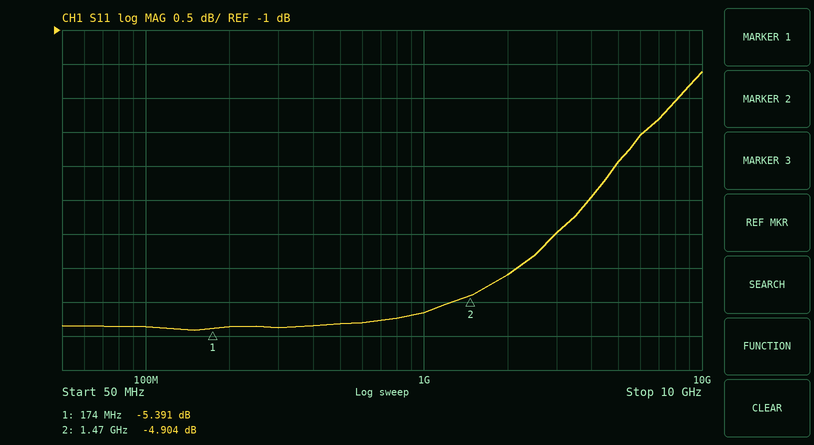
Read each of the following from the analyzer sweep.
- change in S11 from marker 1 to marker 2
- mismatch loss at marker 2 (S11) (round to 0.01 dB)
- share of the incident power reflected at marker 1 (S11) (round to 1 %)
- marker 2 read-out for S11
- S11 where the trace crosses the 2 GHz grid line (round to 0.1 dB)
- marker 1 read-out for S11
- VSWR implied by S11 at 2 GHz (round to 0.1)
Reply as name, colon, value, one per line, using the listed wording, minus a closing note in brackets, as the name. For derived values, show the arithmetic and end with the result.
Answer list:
change in S11 from marker 1 to marker 2: -4.904 − (-5.391) = 0.487 dB
mismatch loss at marker 2 (S11): −10 log10(1 − 10^(-4.904/10)) ≈ 1.70 dB
share of the incident power reflected at marker 1 (S11): 10^(-5.391/10) ≈ 29 %
marker 2 read-out for S11: -4.904 dB
S11 where the trace crosses the 2 GHz grid line: -4.6 dB
marker 1 read-out for S11: -5.391 dB
VSWR implied by S11 at 2 GHz: |Γ| = 10^(-4.6/20) = 0.5888; VSWR = (1 + 0.5888)/(1 − 0.5888) ≈ 3.9
